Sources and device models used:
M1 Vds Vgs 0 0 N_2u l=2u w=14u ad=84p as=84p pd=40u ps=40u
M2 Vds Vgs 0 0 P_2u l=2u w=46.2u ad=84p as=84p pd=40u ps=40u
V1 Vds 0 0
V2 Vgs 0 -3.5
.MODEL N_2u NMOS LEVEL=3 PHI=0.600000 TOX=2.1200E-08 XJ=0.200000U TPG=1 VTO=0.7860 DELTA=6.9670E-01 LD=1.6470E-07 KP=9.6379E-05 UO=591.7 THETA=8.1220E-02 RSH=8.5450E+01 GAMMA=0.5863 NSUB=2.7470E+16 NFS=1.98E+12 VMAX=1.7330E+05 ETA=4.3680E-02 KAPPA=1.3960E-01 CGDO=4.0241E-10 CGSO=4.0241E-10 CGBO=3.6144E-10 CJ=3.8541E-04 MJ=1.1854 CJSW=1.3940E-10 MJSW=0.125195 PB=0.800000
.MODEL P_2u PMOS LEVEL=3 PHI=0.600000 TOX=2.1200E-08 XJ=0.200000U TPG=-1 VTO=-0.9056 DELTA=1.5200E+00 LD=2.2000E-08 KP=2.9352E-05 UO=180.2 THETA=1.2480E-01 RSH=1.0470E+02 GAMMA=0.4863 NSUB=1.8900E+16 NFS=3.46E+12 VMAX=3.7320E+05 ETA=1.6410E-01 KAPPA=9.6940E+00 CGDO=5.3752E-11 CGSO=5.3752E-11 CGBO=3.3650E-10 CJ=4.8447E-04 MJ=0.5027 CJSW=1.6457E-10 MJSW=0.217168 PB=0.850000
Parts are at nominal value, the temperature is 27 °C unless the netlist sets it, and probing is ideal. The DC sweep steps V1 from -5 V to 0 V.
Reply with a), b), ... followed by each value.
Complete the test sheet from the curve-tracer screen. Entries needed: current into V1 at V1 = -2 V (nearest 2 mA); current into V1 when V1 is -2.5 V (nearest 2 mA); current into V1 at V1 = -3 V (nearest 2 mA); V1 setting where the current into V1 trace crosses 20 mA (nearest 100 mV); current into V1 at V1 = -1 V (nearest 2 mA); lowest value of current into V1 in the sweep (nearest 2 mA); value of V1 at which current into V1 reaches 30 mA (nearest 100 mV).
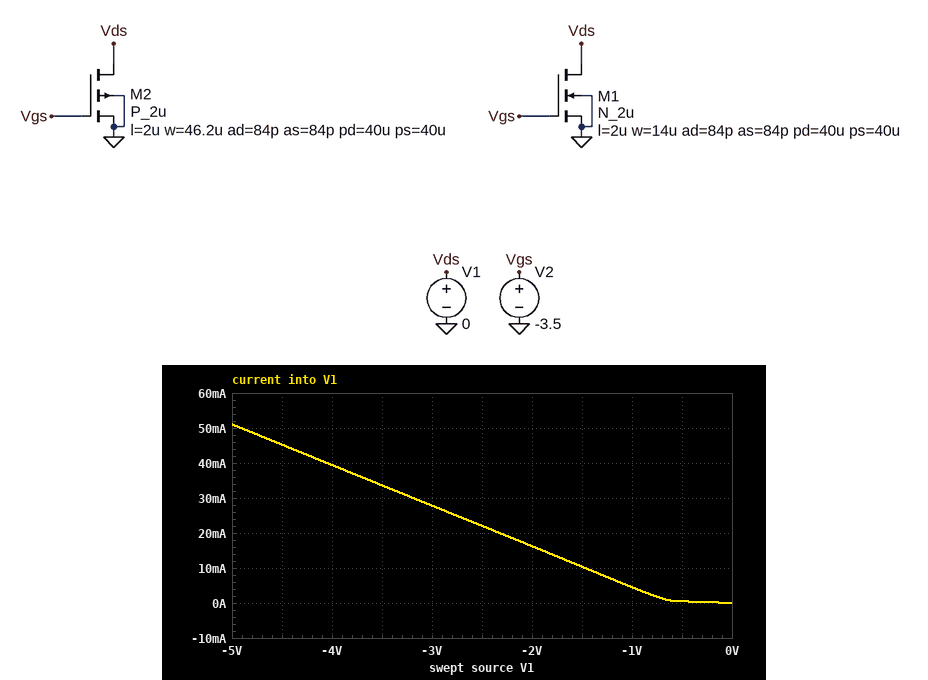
a) 16 mA
b) 22 mA
c) 28 mA
d) -2.3 V
e) 4 mA
f) 0 A
g) -3.2 V
